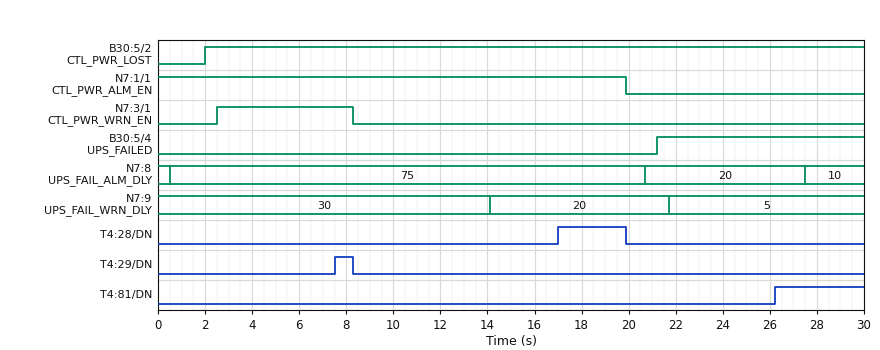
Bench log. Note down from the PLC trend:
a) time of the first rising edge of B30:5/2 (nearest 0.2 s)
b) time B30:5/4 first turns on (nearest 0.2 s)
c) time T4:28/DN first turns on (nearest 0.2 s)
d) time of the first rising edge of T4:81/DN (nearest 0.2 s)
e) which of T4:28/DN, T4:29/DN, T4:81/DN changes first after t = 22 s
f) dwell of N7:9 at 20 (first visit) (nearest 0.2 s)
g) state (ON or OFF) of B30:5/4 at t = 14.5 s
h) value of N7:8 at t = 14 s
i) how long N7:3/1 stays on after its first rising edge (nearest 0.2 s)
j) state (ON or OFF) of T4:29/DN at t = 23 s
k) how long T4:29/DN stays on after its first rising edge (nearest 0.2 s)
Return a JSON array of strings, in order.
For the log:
["2.0 s", "21.2 s", "17.0 s", "26.2 s", "T4:81/DN", "7.6 s", "OFF", "75", "5.8 s", "OFF", "0.8 s"]
